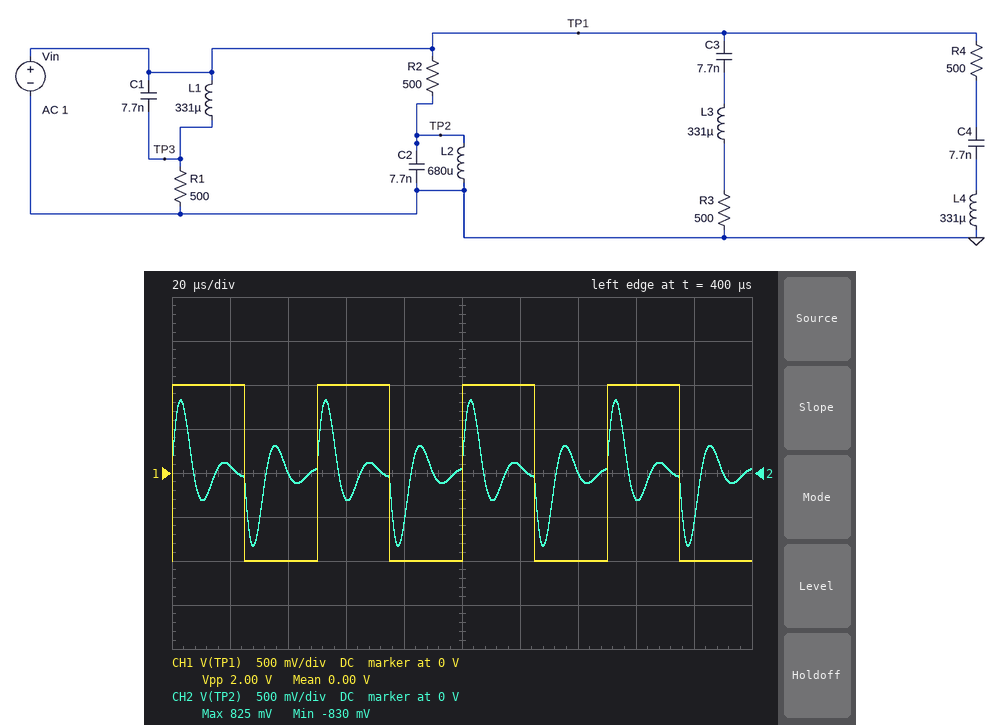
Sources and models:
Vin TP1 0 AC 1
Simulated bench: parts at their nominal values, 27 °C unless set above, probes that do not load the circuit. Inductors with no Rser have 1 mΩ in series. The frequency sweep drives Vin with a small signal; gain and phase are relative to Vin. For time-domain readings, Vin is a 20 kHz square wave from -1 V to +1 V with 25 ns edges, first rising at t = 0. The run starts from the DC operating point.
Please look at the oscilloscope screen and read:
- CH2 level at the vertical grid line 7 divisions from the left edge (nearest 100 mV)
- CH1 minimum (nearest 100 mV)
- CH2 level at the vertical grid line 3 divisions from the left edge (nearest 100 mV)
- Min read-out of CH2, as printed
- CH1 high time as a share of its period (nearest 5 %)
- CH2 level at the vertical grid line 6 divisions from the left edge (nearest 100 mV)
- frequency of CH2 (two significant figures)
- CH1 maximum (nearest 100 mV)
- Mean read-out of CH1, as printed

0 V
-1.0 V
-300 mV
-830 mV
50 %
100 mV
20 kHz
1.0 V
0.00 V
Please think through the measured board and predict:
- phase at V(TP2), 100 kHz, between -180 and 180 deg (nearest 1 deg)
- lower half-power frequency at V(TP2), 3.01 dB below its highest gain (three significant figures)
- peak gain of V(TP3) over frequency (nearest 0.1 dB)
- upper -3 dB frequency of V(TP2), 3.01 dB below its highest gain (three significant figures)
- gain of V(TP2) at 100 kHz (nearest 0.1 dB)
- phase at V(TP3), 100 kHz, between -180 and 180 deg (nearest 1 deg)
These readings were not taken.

-51 deg
51.9 kHz
0 dB
93.2 kHz
-4.1 dB
89 deg
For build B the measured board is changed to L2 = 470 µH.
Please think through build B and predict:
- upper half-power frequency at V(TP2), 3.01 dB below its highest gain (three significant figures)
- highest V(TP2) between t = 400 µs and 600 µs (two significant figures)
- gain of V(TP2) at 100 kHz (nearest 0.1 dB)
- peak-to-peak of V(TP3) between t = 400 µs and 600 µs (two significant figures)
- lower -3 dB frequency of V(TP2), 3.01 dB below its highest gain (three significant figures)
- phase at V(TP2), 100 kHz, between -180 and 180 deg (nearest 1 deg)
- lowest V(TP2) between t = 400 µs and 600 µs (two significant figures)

107 kHz
680 mV
-1.8 dB
2.7 V
65.5 kHz
-36 deg
-680 mV
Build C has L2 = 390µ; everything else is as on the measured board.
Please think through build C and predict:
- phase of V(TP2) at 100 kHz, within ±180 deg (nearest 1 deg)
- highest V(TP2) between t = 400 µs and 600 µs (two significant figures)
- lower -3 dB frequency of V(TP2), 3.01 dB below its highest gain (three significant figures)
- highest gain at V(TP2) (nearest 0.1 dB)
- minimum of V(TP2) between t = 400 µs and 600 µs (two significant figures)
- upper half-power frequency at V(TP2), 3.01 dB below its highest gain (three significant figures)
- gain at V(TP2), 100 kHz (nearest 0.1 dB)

-21 deg
650 mV
73.5 kHz
0 dB
-650 mV
115 kHz
-0.6 dB
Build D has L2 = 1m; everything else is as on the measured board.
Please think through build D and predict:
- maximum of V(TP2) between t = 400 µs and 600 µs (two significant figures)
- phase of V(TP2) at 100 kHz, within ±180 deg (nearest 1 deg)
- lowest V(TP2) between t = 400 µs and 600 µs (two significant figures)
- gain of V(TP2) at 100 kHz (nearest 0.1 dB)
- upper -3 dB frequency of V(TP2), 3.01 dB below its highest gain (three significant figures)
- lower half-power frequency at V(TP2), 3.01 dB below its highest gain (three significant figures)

910 mV
-58 deg
-910 mV
-5.6 dB
81.6 kHz
40.3 kHz
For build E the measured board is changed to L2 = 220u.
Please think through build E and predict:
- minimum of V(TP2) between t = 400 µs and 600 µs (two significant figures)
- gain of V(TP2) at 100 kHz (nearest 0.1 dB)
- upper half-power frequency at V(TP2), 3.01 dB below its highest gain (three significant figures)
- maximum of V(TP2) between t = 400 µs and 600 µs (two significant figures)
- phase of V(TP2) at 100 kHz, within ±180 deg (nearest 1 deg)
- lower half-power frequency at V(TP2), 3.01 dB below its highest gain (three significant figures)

-510 mV
-3.9 dB
145 kHz
510 mV
50 deg
103 kHz
